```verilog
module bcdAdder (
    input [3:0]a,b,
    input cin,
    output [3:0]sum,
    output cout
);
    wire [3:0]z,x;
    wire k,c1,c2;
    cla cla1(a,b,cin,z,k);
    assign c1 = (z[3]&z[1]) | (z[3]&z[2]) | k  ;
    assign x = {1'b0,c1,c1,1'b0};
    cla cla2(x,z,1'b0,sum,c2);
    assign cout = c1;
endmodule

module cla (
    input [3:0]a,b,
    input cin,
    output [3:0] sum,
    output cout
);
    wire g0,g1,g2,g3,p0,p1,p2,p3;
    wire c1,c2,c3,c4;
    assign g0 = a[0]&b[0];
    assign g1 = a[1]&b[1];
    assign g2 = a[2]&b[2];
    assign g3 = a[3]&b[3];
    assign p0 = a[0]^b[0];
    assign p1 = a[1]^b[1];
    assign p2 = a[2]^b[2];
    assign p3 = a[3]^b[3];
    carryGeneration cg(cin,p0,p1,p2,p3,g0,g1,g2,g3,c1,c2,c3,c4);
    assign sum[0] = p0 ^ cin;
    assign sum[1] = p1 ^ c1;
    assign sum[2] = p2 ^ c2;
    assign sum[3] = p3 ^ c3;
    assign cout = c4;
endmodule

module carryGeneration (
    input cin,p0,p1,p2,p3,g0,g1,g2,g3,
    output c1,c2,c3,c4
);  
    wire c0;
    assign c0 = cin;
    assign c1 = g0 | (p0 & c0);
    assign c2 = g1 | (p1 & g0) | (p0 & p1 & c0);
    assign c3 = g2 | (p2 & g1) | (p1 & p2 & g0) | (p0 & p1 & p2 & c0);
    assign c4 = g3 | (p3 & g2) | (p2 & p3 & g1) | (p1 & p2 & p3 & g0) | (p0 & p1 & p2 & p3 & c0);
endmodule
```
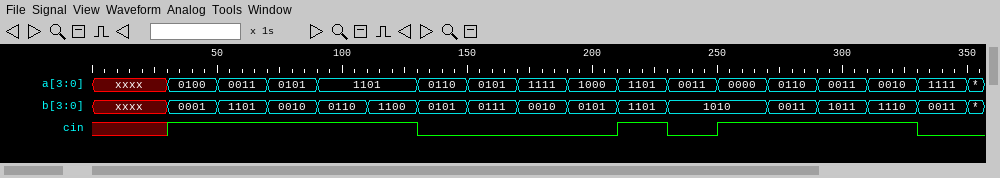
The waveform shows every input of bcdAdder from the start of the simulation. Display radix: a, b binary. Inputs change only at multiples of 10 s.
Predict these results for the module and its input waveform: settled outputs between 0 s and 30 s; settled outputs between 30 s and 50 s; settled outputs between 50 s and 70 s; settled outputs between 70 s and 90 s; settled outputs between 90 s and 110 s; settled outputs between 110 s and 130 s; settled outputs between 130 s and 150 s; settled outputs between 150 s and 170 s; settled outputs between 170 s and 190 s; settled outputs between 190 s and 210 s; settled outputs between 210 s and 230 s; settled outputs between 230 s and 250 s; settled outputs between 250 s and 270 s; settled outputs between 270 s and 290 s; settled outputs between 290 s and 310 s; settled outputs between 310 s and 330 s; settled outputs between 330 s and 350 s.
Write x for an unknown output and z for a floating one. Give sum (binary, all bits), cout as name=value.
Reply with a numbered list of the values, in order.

1. sum=x, cout=x
2. sum=0110, cout=0
3. sum=0111, cout=1
4. sum=1000, cout=0
5. sum=1010, cout=1
6. sum=0000, cout=1
7. sum=0001, cout=1
8. sum=0010, cout=1
9. sum=0111, cout=1
10. sum=0011, cout=1
11. sum=0001, cout=1
12. sum=0011, cout=1
13. sum=0001, cout=1
14. sum=0000, cout=1
15. sum=0101, cout=1
16. sum=0111, cout=1
17. sum=1000, cout=1
